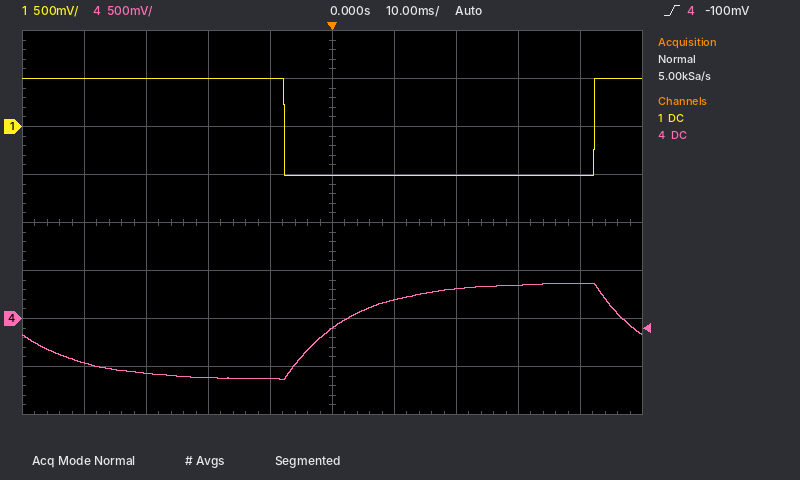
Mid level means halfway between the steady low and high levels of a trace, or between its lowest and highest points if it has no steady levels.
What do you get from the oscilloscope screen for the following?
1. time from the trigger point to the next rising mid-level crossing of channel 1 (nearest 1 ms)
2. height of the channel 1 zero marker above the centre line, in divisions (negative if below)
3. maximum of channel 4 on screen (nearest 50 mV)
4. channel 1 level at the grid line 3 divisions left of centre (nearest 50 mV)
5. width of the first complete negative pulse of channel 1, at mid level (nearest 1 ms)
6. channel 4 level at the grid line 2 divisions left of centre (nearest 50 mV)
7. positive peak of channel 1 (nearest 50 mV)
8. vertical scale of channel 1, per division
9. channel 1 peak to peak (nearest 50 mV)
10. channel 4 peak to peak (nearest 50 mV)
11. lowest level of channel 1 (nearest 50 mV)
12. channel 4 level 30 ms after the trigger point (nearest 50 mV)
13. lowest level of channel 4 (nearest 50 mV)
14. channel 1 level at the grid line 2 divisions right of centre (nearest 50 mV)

42 ms
+2.0 div
350 mV
500 mV
50 ms
-600 mV
500 mV
500 mV
1.00 V
1.00 V
-500 mV
350 mV
-650 mV
-500 mV
